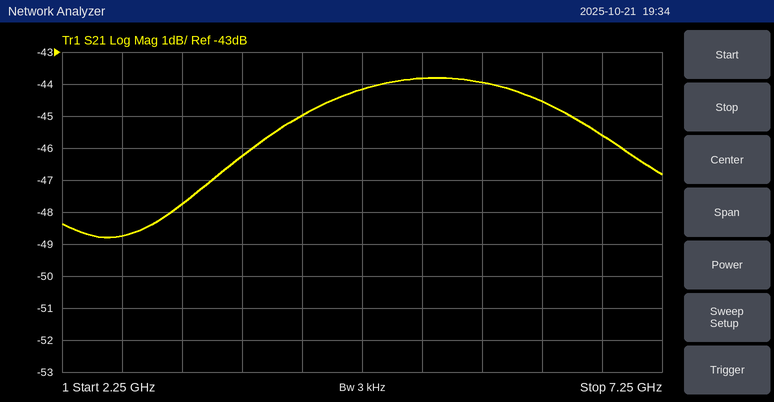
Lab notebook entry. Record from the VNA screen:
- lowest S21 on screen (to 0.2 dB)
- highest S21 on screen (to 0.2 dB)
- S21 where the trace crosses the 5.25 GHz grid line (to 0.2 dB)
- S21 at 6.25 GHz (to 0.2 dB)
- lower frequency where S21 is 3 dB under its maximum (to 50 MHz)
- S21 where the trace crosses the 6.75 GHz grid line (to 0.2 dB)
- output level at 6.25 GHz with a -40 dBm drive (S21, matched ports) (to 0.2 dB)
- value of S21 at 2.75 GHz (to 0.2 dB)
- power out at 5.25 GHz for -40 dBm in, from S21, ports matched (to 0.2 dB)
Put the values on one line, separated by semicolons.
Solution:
-48.8 dB; -43.8 dB; -43.8 dB; -44.6 dB; 3.55 GHz; -45.6 dB; -84.6 dBm; -48.8 dB; -83.8 dBm
